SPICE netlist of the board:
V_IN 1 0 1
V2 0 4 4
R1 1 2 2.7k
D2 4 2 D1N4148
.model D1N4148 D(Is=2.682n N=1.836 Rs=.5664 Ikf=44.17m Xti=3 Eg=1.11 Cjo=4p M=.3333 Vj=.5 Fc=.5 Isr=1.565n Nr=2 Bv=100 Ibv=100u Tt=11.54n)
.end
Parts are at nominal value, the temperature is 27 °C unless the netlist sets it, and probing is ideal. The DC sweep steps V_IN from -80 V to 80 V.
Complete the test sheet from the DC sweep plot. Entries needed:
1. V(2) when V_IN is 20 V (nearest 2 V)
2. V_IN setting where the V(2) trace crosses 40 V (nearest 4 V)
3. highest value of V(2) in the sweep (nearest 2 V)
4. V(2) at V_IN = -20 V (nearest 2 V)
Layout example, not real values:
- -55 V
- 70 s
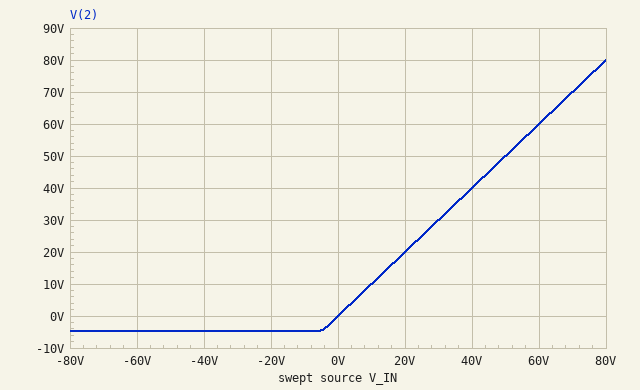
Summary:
- 20 V
- 40 V
- 80 V
- -4 V
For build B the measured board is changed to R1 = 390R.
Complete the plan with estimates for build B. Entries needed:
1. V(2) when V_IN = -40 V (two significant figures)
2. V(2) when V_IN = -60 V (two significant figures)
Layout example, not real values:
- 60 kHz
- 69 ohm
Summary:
- -4.9 V
- -5.0 V
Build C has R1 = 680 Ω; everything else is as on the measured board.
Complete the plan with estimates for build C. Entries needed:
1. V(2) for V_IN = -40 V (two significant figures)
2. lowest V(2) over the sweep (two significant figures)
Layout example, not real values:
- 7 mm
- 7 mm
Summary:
- -4.9 V
- -5.0 V
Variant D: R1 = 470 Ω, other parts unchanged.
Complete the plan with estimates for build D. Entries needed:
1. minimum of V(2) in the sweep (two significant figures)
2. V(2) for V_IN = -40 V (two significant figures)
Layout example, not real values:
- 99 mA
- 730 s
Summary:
- -5.0 V
- -4.9 V
